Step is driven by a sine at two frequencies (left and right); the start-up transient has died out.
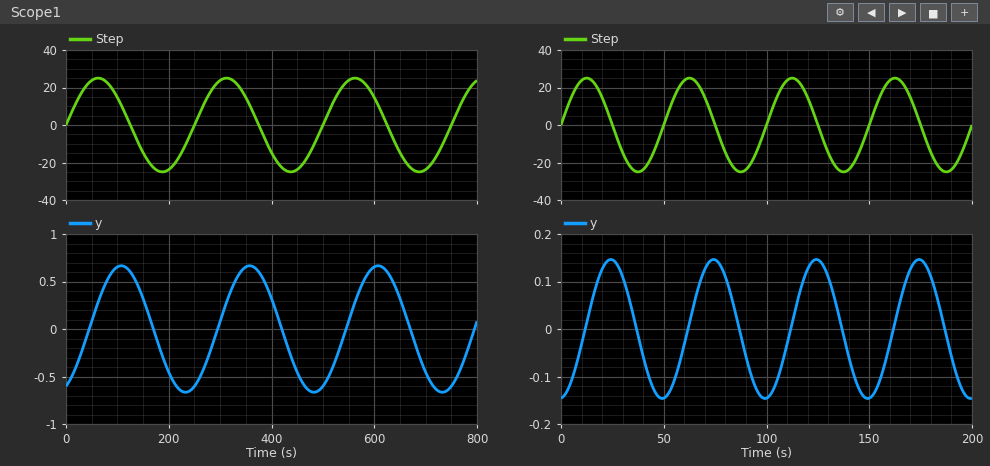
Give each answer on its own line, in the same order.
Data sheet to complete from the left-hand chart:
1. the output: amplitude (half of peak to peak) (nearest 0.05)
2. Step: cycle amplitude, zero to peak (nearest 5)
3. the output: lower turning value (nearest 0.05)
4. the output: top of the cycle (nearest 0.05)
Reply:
0.65
25
-0.65
0.65
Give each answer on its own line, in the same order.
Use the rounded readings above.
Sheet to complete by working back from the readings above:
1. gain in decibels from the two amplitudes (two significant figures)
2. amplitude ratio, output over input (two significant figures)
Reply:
-32 dB
0.026
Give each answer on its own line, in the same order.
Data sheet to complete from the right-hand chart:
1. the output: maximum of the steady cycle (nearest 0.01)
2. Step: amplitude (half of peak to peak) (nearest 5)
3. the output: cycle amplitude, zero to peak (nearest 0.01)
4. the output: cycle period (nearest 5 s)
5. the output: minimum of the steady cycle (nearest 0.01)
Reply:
0.15
25
0.15
50 s
-0.15
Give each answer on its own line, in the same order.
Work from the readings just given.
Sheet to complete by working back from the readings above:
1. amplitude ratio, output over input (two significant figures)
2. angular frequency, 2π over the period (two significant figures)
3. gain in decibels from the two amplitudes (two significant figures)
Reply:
0.0060
0.13 rad/s
-44 dB
